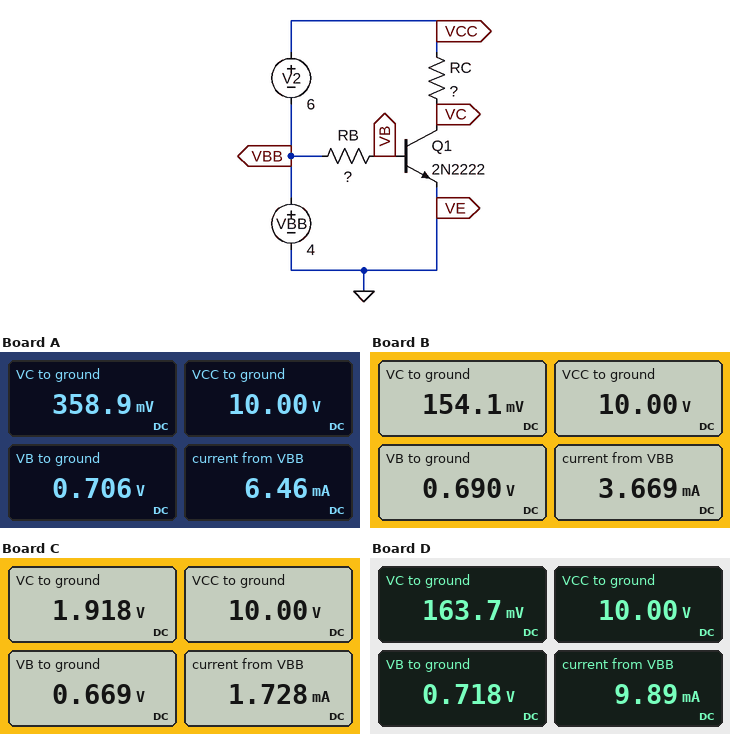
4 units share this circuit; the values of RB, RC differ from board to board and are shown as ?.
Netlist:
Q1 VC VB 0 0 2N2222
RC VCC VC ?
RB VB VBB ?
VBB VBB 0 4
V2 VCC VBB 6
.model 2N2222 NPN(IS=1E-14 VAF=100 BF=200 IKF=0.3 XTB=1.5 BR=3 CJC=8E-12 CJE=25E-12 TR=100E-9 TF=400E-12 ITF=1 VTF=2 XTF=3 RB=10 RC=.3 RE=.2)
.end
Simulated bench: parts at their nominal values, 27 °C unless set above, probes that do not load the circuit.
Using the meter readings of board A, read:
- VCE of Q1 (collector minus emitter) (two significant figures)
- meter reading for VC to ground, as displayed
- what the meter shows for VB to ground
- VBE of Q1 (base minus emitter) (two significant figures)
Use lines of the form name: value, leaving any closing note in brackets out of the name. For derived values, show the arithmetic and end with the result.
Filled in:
VCE of Q1 (collector minus emitter): 358.9 mV = 360 mV
meter reading for VC to ground, as displayed: 358.9 mV
what the meter shows for VB to ground: 0.706 V
VBE of Q1 (base minus emitter): 706 mV = 710 mV
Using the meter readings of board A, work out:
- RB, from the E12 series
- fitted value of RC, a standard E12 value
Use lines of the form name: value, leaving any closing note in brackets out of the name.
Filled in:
RB, from the E12 series: 100 kΩ
fitted value of RC, a standard E12 value: 1.5 kΩ
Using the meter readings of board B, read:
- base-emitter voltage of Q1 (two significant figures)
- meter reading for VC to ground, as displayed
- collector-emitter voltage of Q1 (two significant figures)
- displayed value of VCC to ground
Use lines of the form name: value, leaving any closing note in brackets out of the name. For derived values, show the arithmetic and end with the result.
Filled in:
base-emitter voltage of Q1: 690 mV = 690 mV
meter reading for VC to ground, as displayed: 154.1 mV
collector-emitter voltage of Q1: 154.1 mV = 150 mV
displayed value of VCC to ground: 10.00 V
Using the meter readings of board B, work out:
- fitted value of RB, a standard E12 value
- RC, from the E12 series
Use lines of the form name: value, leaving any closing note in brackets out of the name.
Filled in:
fitted value of RB, a standard E12 value: 150 kΩ
RC, from the E12 series: 2.7 kΩ
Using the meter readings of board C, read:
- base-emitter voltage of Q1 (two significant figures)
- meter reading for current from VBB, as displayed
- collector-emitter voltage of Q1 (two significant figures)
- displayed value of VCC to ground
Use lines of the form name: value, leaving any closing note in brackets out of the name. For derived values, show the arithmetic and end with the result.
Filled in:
base-emitter voltage of Q1: 669 mV = 670 mV
meter reading for current from VBB, as displayed: 1.728 mA
collector-emitter voltage of Q1: 1.918 V = 1.9 V
displayed value of VCC to ground: 10.00 V
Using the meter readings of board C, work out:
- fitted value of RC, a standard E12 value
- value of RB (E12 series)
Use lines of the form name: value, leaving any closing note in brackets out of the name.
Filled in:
fitted value of RC, a standard E12 value: 4.7 kΩ
value of RB: 390 kΩ
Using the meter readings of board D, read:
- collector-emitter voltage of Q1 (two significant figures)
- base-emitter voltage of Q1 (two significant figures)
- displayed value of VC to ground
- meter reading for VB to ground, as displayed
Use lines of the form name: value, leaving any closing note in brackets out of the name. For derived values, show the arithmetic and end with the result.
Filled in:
collector-emitter voltage of Q1: 163.7 mV = 160 mV
base-emitter voltage of Q1: 718 mV = 720 mV
displayed value of VC to ground: 163.7 mV
meter reading for VB to ground, as displayed: 0.718 V
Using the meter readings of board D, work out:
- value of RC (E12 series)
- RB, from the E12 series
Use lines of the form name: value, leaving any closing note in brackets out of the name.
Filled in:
value of RC: 1 kΩ
RB, from the E12 series: 56 kΩ
